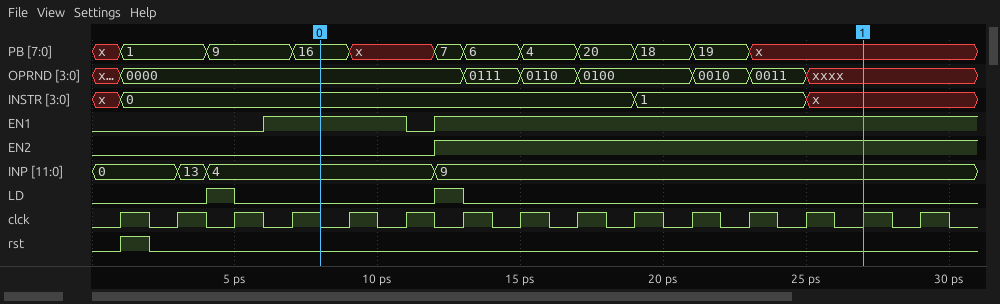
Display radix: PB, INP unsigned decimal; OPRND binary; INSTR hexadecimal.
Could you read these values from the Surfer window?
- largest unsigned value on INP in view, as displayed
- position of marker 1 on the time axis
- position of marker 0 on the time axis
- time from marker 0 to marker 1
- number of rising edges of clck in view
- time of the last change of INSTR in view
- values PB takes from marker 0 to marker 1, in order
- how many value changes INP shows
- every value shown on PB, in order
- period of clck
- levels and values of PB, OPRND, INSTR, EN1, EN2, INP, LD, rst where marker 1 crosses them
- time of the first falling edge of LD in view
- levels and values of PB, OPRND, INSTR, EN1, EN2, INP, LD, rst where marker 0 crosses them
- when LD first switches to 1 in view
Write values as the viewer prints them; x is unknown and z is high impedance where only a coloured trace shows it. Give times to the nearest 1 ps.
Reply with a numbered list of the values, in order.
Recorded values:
1. 13
2. 27 ps
3. 8 ps
4. 19 ps
5. 15
6. 25 ps
7. 16, x, 7, 6, 4, 20, 18, 19, x
8. 3
9. x, 1, 9, 16, x, 7, 6, 4, 20, 18, 19, x
10. 2 ps
11. PB=x, OPRND=xxxx, INSTR=x, EN1=1, EN2=1, INP=9, LD=0, rst=0
12. 5 ps
13. PB=16, OPRND=0000, INSTR=0, EN1=1, EN2=0, INP=4, LD=0, rst=0
14. 4 ps
